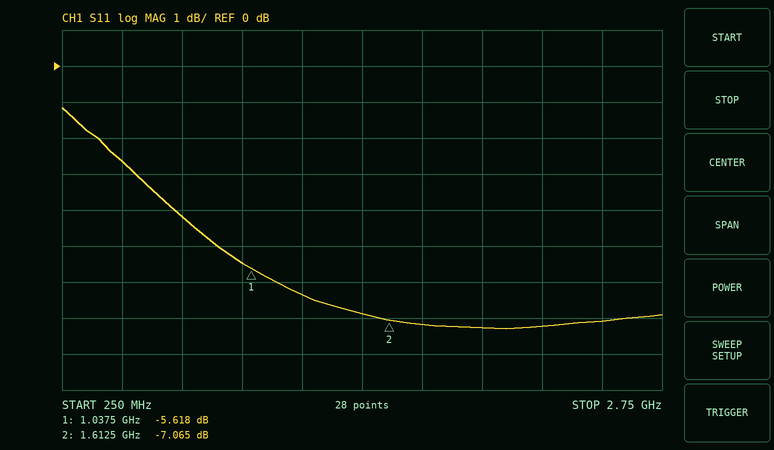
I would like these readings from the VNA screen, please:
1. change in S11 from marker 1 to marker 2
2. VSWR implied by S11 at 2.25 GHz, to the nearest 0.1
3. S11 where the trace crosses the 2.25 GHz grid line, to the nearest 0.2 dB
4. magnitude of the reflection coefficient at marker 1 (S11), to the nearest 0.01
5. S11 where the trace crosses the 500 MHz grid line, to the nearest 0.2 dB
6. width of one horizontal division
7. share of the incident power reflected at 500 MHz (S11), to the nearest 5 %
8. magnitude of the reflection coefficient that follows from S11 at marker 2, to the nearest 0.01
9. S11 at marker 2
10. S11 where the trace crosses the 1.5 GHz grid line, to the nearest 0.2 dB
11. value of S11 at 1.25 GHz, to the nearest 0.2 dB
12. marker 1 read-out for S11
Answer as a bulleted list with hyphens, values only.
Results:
- -1.447 dB
- 2.5
- -7.2 dB
- 0.52
- -2.6 dB
- 250 MHz
- 55 %
- 0.44
- -7.065 dB
- -6.8 dB
- -6.4 dB
- -5.618 dB
